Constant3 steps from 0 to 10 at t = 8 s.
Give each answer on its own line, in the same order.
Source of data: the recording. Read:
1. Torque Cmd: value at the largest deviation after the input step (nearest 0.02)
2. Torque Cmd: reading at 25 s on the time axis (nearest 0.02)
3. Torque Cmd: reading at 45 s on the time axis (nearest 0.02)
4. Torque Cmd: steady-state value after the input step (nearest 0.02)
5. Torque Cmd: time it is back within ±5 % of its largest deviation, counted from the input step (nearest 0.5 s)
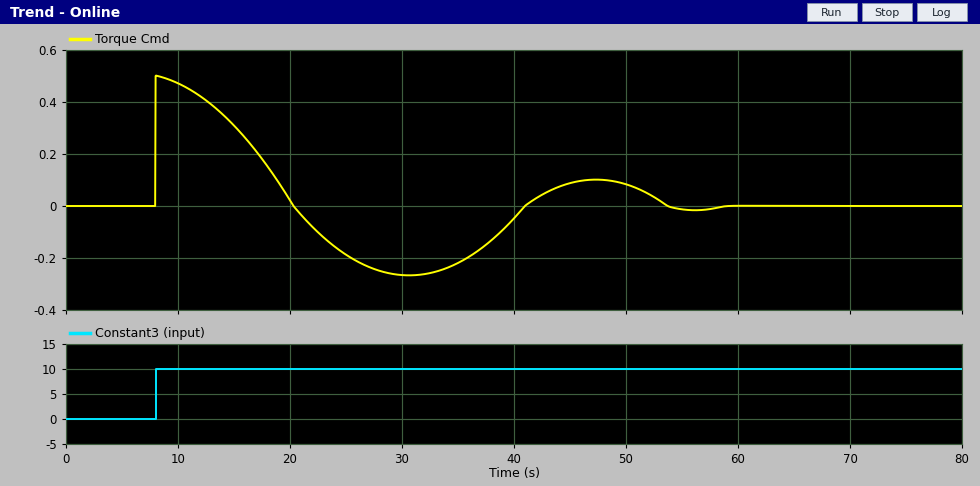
0.50
-0.18
0.08
0.00
45.0 s
